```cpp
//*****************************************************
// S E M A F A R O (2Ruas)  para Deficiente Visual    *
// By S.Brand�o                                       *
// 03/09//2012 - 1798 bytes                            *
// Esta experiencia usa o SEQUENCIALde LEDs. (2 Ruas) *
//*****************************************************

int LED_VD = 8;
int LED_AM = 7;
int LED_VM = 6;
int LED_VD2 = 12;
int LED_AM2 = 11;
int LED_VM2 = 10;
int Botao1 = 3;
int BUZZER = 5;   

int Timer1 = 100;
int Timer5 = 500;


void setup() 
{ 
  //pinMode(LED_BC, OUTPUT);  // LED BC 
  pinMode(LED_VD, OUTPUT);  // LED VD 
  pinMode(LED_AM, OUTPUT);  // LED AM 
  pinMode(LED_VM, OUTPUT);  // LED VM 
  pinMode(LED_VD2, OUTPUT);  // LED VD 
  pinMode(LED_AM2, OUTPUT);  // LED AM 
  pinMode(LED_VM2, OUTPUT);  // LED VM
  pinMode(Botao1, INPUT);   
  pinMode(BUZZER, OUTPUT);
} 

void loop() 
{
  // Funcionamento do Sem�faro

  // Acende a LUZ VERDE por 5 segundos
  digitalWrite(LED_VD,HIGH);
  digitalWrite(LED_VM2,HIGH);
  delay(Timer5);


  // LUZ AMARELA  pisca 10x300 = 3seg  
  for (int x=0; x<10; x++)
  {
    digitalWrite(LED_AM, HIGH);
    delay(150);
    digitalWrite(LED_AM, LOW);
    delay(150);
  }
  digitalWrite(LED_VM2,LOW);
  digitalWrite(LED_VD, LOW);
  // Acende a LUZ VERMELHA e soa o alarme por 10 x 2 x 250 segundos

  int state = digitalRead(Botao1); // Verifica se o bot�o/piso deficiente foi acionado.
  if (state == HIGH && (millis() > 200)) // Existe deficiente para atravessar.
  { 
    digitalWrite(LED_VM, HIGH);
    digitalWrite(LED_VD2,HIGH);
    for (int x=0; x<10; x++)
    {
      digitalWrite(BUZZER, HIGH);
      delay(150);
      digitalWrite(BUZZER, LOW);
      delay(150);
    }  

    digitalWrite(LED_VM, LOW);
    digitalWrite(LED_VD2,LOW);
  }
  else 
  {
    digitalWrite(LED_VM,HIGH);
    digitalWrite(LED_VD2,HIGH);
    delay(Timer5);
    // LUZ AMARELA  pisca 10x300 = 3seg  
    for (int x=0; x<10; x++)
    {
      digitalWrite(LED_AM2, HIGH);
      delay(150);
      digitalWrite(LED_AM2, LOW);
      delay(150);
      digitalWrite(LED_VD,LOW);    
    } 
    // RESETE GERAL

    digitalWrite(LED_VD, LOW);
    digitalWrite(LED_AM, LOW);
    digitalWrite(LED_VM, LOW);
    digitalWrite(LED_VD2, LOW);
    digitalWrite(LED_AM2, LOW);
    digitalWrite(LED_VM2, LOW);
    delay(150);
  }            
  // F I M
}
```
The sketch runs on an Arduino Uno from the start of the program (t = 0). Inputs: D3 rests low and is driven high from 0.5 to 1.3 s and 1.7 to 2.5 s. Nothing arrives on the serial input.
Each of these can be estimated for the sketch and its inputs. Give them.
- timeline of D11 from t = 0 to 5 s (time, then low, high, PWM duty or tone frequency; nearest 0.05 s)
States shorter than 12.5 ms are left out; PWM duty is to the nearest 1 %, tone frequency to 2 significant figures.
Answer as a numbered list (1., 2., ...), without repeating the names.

1. 0 s low; 4 s high; 4.15 s low; 4.3 s high; 4.45 s low; 4.6 s high; 4.75 s low; 4.9 s high
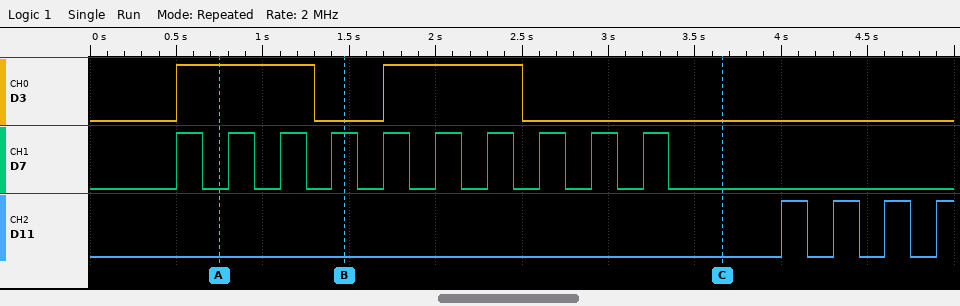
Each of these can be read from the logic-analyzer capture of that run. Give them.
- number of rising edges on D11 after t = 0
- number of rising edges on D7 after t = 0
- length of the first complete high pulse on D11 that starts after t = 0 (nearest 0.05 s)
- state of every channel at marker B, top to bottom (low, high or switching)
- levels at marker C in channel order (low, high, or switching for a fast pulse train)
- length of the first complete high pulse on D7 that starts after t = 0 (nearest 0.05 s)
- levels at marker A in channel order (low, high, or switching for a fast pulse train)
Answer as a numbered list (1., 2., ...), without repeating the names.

1. 4
2. 10
3. 0.15 s
4. D3 low, D7 high, D11 low
5. D3 low, D7 low, D11 low
6. 0.15 s
7. D3 high, D7 low, D11 low
